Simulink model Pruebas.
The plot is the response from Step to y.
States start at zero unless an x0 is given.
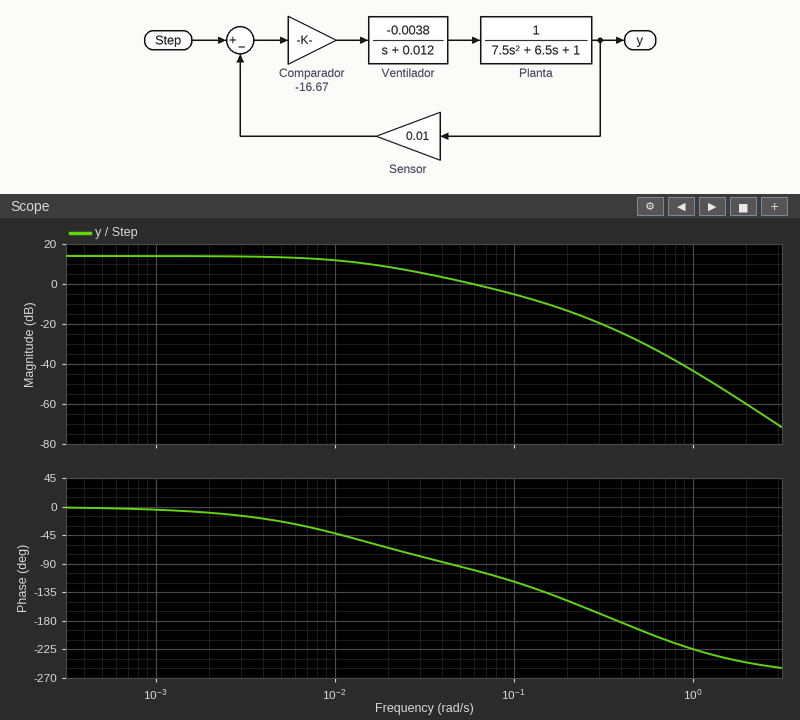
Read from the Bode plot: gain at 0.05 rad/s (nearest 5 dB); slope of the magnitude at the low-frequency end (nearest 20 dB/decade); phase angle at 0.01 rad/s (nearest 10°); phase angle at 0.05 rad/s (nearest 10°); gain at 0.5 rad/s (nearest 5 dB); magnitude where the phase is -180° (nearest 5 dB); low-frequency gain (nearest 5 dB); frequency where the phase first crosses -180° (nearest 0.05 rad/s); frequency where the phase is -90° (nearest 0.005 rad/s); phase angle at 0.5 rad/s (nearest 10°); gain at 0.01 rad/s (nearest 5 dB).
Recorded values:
0 dB
0 dB/decade
-40°
-90°
-30 dB
-25 dB
15 dB
0.40 rad/s
0.045 rad/s
-190°
10 dB
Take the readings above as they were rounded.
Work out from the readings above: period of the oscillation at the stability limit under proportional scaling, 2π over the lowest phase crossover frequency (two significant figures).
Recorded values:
16 s
